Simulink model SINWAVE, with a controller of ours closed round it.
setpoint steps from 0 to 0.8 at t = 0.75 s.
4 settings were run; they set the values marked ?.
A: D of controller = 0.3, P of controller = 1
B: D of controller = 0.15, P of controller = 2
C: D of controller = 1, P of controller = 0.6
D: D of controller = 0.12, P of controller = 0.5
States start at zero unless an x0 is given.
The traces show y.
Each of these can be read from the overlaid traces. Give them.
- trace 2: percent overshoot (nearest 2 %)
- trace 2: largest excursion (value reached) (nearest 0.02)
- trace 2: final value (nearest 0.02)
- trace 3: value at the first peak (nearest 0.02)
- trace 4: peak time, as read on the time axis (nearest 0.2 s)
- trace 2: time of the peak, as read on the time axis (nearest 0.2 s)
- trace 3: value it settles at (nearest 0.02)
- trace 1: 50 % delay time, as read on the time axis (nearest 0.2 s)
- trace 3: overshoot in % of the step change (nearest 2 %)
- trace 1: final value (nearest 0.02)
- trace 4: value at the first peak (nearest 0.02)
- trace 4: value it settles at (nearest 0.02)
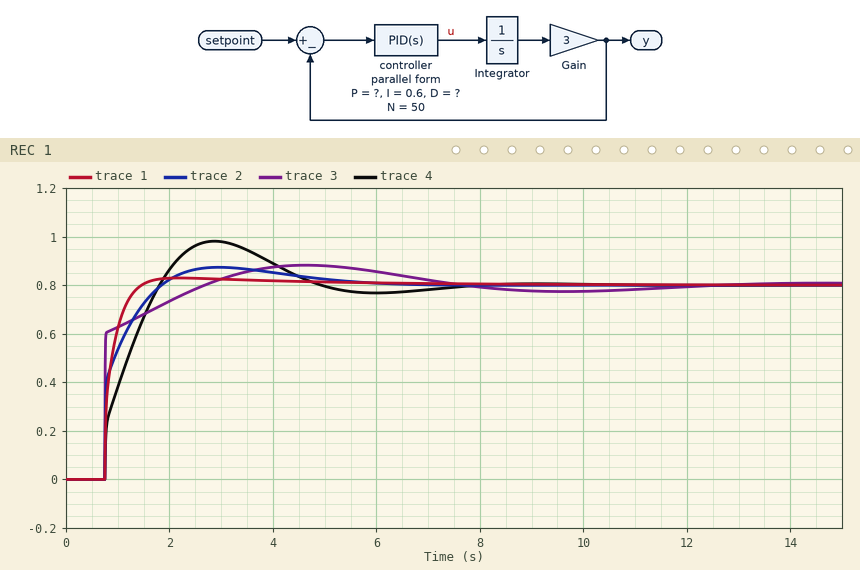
10 %
0.88
0.80
0.88
2.8 s
3.0 s
0.80
0.8 s
10 %
0.80
0.98
0.80
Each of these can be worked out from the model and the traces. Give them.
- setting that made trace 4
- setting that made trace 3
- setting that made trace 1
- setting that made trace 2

D
C
B
A
